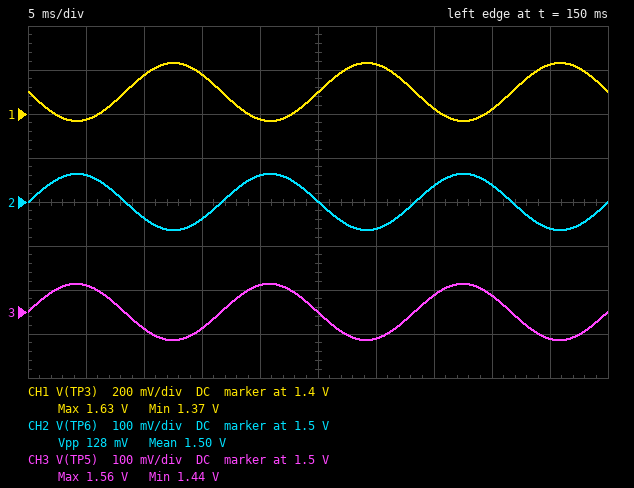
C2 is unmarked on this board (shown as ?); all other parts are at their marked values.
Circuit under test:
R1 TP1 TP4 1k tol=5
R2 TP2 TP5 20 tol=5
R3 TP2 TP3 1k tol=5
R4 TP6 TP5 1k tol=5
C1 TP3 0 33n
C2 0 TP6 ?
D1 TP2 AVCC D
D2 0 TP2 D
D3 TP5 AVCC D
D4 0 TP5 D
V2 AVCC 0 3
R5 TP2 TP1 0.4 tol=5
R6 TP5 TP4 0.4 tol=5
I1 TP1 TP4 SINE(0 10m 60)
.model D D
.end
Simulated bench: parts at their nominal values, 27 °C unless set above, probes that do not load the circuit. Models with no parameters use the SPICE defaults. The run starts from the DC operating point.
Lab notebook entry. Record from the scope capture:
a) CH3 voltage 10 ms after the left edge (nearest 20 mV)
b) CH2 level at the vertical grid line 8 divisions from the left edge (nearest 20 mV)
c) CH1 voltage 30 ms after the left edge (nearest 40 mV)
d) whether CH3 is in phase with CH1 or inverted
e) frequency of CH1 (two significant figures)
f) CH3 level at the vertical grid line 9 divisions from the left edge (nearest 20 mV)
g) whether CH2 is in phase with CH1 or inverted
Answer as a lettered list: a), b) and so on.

a) 1.46 V
b) 1.54 V
c) 1.64 V
d) inverted
e) 60 Hz
f) 1.44 V
g) inverted
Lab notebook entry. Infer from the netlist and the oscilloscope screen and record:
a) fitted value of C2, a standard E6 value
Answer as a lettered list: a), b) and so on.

a) 68 nF
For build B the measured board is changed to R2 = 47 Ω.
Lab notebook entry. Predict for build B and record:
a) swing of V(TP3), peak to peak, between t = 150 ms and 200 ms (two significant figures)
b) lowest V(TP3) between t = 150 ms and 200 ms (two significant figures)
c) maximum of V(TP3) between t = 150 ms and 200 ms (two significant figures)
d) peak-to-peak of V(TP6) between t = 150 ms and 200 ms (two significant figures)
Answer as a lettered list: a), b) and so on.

a) 600 mV
b) 1.2 V
c) 1.8 V
d) 290 mV
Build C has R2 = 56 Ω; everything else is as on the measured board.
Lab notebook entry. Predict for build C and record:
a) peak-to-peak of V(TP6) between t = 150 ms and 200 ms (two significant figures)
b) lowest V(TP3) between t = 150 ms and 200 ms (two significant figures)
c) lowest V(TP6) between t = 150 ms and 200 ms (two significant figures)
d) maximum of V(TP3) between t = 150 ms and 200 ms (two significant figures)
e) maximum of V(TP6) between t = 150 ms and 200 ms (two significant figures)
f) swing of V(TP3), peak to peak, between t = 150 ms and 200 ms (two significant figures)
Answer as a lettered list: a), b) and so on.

a) 350 mV
b) 1.1 V
c) 1.3 V
d) 1.9 V
e) 1.7 V
f) 710 mV
